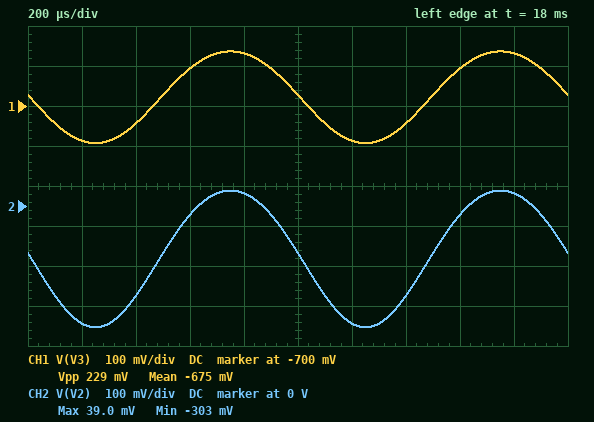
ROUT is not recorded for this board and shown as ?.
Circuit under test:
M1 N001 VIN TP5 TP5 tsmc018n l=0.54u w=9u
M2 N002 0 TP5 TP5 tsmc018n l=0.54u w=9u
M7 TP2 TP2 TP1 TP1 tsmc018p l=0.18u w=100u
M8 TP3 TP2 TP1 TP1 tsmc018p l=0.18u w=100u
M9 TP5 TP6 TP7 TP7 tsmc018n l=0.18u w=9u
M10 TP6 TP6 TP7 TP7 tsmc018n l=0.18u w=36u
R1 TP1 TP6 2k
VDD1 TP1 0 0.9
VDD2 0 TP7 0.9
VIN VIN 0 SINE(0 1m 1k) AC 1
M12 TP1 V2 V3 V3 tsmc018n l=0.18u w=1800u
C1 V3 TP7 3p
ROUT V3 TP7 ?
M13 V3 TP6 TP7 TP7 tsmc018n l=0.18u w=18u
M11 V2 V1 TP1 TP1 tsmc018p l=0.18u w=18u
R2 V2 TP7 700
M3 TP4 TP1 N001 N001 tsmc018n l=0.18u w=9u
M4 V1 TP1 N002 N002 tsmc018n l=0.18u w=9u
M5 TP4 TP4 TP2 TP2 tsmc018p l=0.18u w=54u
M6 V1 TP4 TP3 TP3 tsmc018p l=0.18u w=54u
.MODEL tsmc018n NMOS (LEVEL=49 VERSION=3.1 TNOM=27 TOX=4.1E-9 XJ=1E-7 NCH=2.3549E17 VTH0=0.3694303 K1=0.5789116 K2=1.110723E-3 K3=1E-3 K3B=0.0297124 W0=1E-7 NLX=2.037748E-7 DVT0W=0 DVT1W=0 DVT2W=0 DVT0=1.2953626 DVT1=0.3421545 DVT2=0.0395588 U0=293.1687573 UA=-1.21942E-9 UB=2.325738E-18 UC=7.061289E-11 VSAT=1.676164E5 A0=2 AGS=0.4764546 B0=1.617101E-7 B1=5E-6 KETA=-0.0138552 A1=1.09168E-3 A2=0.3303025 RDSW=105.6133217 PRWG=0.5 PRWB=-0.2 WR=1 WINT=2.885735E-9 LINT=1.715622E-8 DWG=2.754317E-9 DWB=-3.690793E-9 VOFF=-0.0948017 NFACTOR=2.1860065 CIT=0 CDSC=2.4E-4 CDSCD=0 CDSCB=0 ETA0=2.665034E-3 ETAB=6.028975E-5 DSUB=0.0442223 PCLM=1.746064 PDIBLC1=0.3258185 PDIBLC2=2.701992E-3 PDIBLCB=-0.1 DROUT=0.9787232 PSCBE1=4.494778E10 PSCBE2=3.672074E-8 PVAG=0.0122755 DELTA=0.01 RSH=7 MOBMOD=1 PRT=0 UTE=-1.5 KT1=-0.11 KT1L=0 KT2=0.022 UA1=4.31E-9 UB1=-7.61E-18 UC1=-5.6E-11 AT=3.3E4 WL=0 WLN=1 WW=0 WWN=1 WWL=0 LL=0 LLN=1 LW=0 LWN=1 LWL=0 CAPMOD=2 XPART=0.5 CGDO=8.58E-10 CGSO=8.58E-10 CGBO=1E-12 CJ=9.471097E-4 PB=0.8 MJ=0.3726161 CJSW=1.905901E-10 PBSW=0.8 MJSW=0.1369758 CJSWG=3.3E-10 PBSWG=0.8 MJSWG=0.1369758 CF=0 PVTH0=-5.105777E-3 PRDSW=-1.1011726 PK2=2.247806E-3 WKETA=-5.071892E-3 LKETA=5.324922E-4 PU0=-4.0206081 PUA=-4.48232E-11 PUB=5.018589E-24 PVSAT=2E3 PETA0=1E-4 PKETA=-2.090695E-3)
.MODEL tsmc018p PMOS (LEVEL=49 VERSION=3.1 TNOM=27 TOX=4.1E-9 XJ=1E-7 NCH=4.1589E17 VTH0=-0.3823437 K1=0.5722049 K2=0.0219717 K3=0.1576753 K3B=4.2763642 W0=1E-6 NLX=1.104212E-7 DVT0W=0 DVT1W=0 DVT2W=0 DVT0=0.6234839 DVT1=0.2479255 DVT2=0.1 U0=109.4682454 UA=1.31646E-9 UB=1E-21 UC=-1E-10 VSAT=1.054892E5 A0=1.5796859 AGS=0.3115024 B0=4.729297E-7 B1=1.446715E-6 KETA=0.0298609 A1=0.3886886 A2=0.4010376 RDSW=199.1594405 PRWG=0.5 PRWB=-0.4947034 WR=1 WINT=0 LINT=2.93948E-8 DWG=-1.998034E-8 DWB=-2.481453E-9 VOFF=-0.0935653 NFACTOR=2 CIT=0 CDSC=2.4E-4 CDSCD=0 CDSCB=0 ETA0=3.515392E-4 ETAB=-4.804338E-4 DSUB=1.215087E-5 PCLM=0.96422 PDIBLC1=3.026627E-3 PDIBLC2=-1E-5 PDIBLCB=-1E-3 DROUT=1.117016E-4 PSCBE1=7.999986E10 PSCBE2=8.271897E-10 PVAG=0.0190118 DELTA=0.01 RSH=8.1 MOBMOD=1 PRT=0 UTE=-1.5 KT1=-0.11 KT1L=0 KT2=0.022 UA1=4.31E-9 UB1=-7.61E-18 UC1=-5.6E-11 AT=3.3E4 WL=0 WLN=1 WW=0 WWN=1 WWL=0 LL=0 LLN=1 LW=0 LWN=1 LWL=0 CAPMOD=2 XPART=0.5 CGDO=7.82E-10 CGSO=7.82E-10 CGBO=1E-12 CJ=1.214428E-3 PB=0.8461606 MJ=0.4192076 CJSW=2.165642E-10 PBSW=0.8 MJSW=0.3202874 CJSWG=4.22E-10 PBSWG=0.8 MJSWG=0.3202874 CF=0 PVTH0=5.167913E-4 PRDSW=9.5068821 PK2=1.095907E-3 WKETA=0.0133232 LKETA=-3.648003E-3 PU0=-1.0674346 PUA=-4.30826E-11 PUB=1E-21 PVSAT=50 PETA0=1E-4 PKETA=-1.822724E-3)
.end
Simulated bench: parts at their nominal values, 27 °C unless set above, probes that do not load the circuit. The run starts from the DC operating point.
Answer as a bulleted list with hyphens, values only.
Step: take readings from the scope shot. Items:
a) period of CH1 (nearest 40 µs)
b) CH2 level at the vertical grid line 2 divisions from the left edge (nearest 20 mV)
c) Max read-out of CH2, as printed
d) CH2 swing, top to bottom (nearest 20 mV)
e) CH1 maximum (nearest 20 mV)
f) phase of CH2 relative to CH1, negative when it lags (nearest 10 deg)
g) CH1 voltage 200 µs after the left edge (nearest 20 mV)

- 1.00 ms
- -220 mV
- 39.0 mV
- 340 mV
- -560 mV
- 0 deg
- -780 mV
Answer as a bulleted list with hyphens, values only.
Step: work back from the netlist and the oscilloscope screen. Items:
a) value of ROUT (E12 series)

- 39 Ω
